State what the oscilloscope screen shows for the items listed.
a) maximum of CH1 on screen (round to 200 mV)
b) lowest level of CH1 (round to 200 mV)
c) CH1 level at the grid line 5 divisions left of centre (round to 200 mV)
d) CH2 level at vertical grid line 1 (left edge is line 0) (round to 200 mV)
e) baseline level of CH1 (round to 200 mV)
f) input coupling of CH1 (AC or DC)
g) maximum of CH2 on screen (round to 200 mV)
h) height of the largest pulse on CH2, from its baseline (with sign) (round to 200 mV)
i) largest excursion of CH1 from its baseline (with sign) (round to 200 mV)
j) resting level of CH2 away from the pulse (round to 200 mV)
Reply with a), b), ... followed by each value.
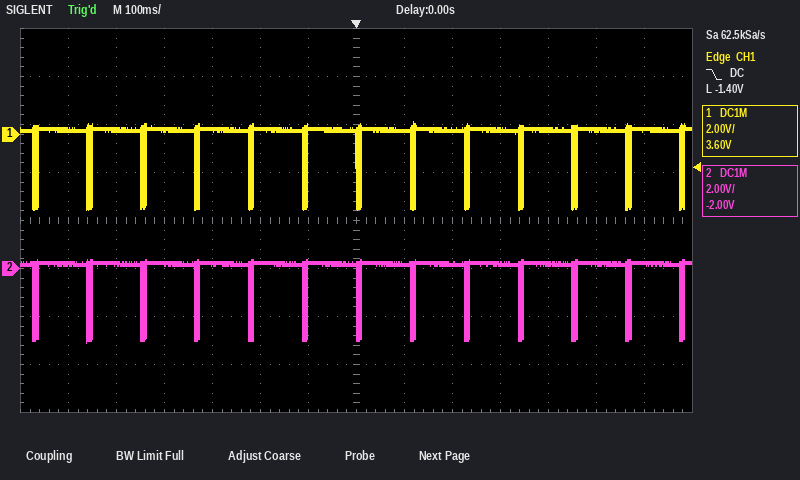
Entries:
a) 600 mV
b) -3.2 V
c) 200 mV
d) 200 mV
e) 200 mV
f) DC
g) 400 mV
h) -3.2 V
i) -3.4 V
j) 200 mV
